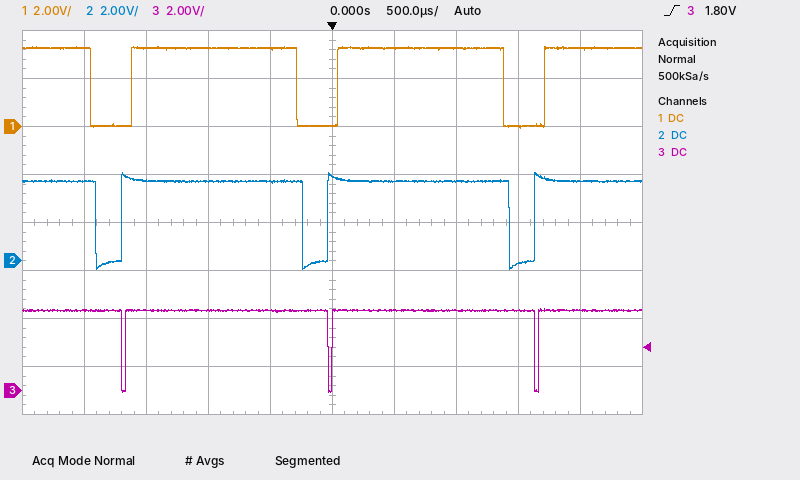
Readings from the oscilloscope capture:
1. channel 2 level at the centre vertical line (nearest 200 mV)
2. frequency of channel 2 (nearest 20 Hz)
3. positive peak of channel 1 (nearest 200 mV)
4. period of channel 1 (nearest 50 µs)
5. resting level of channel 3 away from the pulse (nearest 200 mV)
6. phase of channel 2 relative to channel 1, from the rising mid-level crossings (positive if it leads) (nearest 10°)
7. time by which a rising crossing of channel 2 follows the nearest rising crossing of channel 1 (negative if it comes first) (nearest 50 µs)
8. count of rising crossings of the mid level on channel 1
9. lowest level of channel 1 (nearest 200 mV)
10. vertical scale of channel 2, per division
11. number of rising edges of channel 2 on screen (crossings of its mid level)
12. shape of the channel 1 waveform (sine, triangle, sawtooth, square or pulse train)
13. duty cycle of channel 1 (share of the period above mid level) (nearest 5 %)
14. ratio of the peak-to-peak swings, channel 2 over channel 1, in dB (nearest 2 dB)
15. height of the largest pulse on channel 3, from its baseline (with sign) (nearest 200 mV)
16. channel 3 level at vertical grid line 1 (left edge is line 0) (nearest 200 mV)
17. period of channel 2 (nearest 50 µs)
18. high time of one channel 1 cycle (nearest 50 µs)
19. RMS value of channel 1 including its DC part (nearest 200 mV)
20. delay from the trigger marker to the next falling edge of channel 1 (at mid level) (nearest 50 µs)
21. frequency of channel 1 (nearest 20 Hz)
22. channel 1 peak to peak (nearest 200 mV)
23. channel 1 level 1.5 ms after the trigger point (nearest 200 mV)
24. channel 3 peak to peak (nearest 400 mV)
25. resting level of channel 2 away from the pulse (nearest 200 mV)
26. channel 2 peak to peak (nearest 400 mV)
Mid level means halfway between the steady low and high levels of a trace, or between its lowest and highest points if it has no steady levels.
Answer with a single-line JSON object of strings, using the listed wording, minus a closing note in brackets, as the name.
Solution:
{"channel 2 level at the centre vertical line": "3.6 V", "frequency of channel 2": "600 Hz", "positive peak of channel 1": "3.4 V", "period of channel 1": "1.65 ms", "resting level of channel 3 away from the pulse": "3.4 V", "phase of channel 2 relative to channel 1, from the rising mid-level crossings (positive if it leads)": "+20°", "time by which a rising crossing of channel 2 follows the nearest rising crossing of channel 1 (negative if it comes first)": "-100 µs", "count of rising crossings of the mid level on channel 1": "3", "lowest level of channel 1": "0.0 V", "vertical scale of channel 2, per division": "2 V", "number of rising edges of channel 2 on screen": "3", "shape of the channel 1 waveform": "pulse train", "duty cycle of channel 1 (share of the period above mid level)": "80 %", "ratio of the peak-to-peak swings, channel 2 over channel 1, in dB": "2 dB", "height of the largest pulse on channel 3, from its baseline (with sign)": "-3.4 V", "channel 3 level at vertical grid line 1 (left edge is line 0)": "3.4 V", "period of channel 2": "1.65 ms", "high time of one channel 1 cycle": "1.35 ms", "RMS value of channel 1 including its DC part": "3.0 V", "delay from the trigger marker to the next falling edge of channel 1 (at mid level)": "1.40 ms", "frequency of channel 1": "600 Hz", "channel 1 peak to peak": "3.4 V", "channel 1 level 1.5 ms after the trigger point": "0.0 V", "channel 3 peak to peak": "3.6 V", "resting level of channel 2 away from the pulse": "3.4 V", "channel 2 peak to peak": "4.0 V"}
